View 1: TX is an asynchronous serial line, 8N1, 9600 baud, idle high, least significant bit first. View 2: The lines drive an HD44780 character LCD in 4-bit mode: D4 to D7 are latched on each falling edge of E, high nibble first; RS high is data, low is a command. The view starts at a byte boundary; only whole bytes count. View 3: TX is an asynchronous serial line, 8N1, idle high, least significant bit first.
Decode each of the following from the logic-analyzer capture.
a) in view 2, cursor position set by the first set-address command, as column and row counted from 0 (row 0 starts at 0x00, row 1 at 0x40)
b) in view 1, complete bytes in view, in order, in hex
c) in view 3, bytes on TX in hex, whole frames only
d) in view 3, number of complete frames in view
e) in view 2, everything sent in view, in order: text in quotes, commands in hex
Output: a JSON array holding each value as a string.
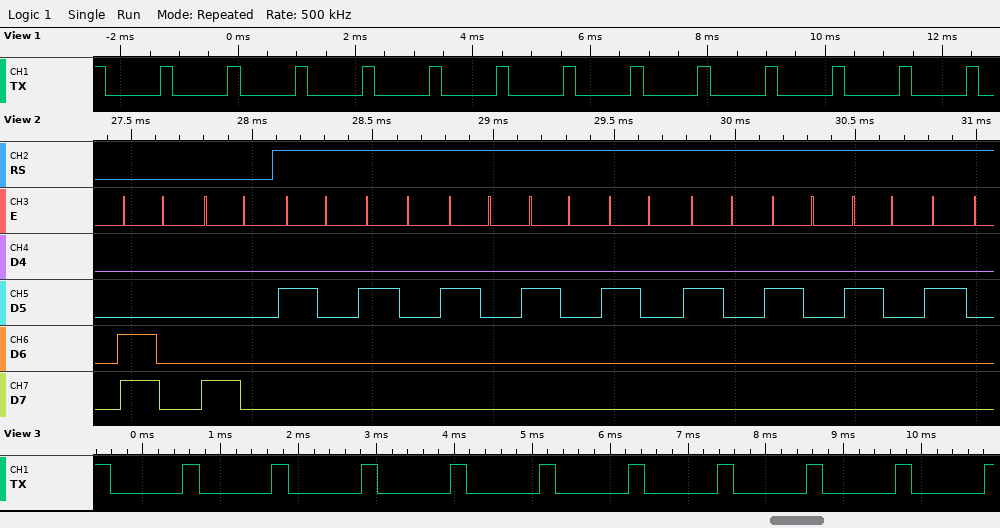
["column 0, row 1", "0x00 0x00 0x00 0x00 0x00 0x00 0x00 0x00 0x00 0x00 0x00 0x00 0x00", "00 00 00 00 00 00 00 00 00 00", "10", "0xC0 0x80 \"         \""]
